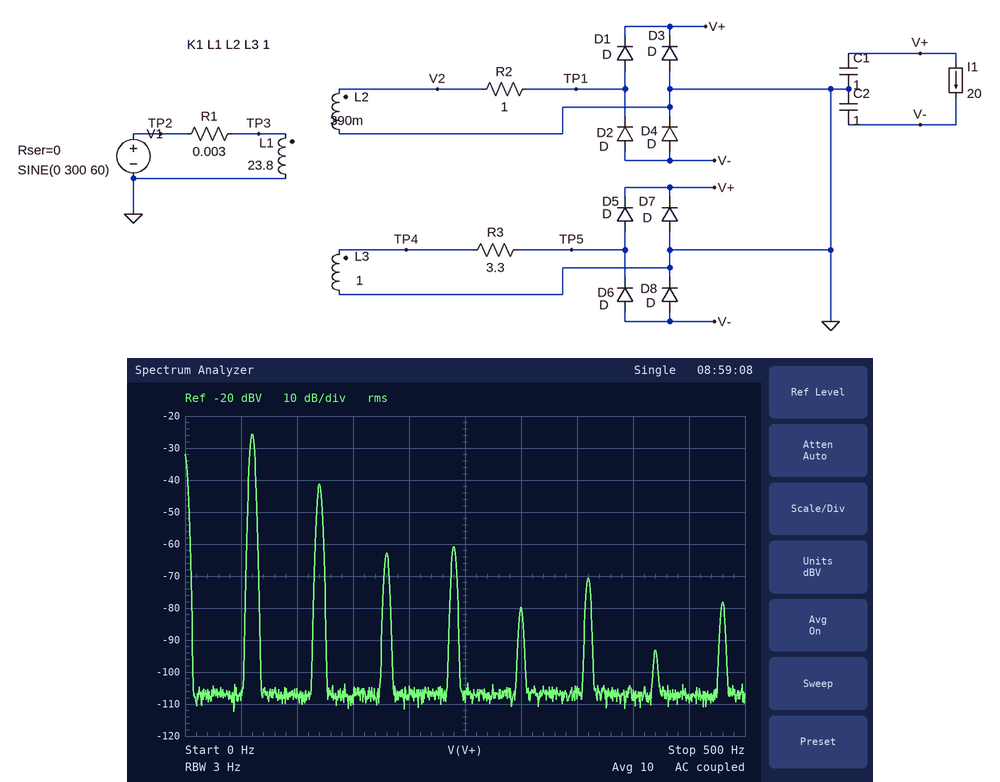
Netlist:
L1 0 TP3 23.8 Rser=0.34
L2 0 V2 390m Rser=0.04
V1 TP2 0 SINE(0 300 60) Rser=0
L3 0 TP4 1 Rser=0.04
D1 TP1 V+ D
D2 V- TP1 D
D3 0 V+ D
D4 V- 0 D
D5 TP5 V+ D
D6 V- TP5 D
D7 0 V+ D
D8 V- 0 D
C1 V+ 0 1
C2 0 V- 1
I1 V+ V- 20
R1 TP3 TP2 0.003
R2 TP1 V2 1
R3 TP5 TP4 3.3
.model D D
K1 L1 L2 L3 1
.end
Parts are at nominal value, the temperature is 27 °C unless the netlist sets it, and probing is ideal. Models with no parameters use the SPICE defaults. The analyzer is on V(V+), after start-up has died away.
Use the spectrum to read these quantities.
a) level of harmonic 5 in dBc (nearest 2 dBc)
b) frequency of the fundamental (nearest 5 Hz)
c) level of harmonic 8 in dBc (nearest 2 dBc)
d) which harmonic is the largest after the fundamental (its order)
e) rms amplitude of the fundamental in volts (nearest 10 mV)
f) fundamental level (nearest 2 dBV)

-54 dBc
60 Hz
-52 dBc
2
50 mV
-26 dBV
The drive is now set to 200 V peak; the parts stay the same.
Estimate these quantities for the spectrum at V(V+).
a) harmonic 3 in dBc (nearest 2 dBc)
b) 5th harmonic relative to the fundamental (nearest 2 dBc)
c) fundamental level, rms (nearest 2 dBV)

-40 dBc
-56 dBc
-30 dBV
